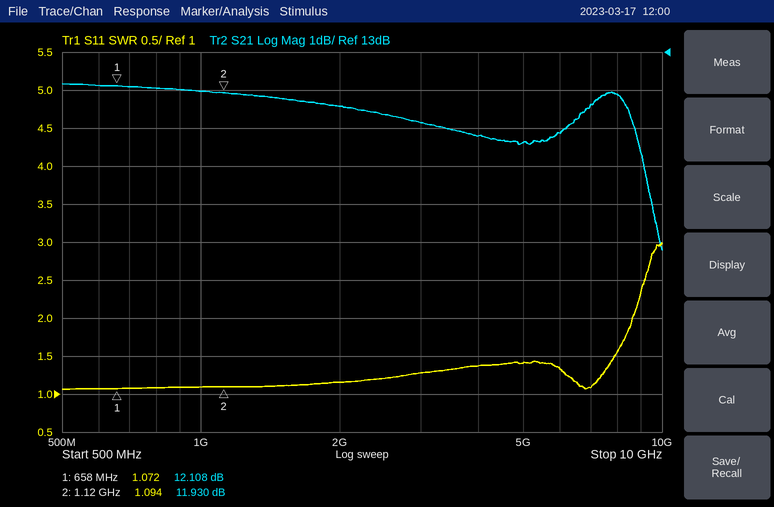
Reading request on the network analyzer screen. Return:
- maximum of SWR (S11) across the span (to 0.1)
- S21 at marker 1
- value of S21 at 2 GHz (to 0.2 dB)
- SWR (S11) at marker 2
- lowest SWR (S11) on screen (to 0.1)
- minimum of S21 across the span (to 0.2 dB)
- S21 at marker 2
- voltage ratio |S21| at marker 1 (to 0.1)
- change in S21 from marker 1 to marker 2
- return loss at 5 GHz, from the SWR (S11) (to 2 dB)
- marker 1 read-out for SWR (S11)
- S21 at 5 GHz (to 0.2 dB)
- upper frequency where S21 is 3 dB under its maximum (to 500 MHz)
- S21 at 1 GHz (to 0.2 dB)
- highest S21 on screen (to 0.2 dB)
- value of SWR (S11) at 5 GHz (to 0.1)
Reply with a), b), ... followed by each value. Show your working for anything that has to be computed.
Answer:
a) 3.0
b) 12.108 dB
c) 11.6 dB
d) 1.094
e) 1.1
f) 7.8 dB
g) 11.930 dB
h) 10^(12.108/20) ≈ 4.0
i) 11.93 − (12.108) = -0.178 dB
j) −20 log10((1.4 − 1)/(1.4 + 1)) ≈ 16 dB
k) 1.072
l) 10.6 dB
m) 9.5 GHz
n) 12.0 dB
o) 12.2 dB
p) 1.4
